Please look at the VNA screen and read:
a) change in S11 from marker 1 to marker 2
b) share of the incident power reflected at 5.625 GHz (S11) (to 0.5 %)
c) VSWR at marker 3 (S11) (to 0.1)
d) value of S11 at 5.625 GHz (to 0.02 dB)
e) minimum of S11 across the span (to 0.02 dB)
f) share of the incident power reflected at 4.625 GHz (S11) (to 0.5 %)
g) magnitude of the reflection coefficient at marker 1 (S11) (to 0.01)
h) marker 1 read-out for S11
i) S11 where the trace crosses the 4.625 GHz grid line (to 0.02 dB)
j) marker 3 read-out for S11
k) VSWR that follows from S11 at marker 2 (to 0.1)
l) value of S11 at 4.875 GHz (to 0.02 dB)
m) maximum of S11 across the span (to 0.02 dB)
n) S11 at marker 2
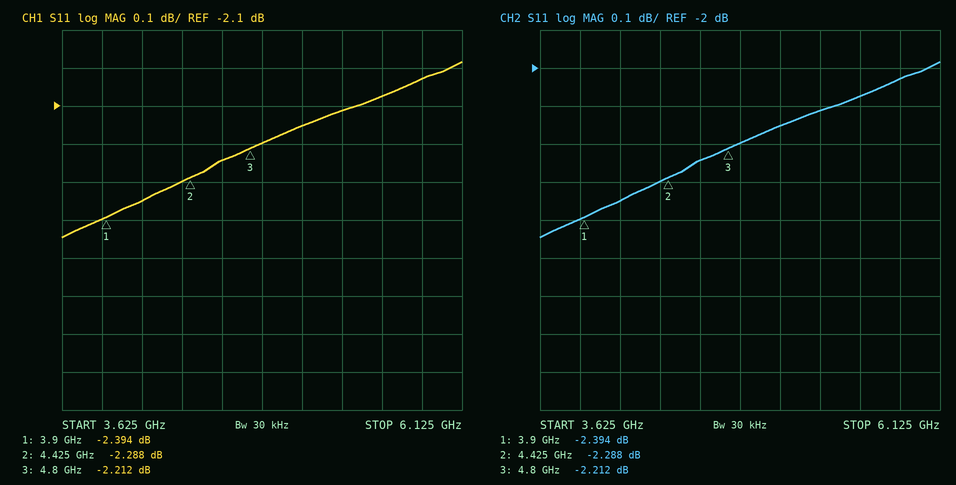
0.106 dB
62.0 %
7.9
-2.08 dB
-2.44 dB
59.5 %
0.76
-2.394 dB
-2.24 dB
-2.212 dB
7.6
-2.20 dB
-1.98 dB
-2.288 dB
